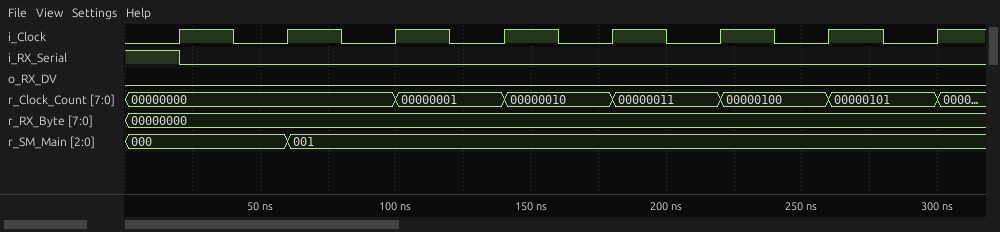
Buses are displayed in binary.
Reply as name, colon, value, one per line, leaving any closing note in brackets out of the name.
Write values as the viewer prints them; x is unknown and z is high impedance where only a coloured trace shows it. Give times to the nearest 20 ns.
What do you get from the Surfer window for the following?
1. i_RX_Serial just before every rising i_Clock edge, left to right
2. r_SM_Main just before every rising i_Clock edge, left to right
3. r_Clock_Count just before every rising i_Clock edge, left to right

i_RX_Serial just before every rising i_Clock edge, left to right: 1 0 0 0 0 0 0 0
r_SM_Main just before every rising i_Clock edge, left to right: 000, 000, 001, 001, 001, 001, 001, 001
r_Clock_Count just before every rising i_Clock edge, left to right: 00000000, 00000000, 00000000, 00000001, 00000010, 00000011, 00000100, 00000101
